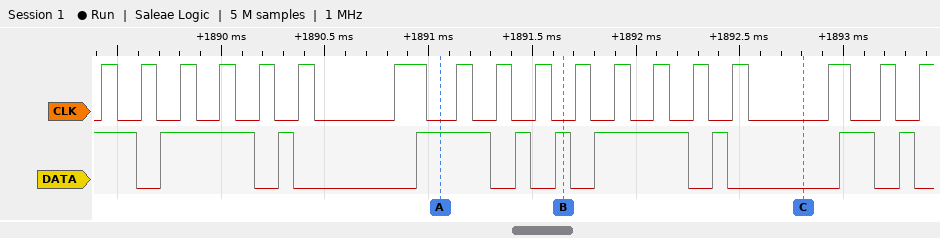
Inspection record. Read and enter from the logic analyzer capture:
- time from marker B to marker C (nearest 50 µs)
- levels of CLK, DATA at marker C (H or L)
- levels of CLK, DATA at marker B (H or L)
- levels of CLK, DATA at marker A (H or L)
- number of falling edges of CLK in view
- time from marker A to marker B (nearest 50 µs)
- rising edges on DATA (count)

1150 µs
CLK=L, DATA=L
CLK=L, DATA=H
CLK=L, DATA=H
17
600 µs
9
